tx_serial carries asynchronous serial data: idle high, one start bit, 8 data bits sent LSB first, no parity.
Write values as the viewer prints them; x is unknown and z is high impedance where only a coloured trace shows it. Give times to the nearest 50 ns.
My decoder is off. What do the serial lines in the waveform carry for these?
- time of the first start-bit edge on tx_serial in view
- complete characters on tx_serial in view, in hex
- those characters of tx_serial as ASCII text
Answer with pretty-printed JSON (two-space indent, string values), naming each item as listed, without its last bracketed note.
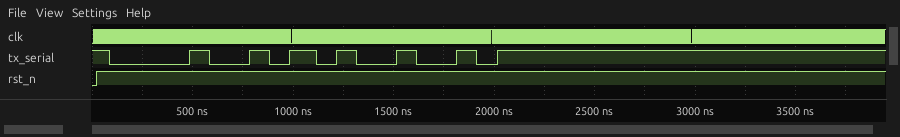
{
  "time of the first start-bit edge on tx_serial in view": "100 ns",
  "complete characters on tx_serial in view, in hex": "48, 49",
  "those characters of tx_serial as ASCII text": "\"HI\""
}
